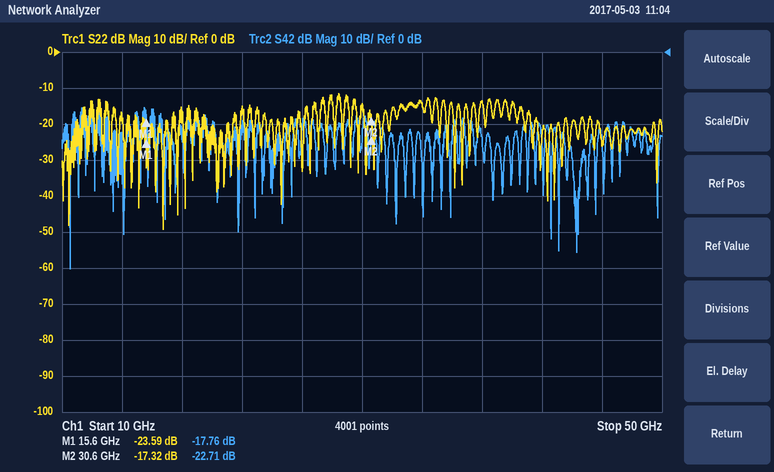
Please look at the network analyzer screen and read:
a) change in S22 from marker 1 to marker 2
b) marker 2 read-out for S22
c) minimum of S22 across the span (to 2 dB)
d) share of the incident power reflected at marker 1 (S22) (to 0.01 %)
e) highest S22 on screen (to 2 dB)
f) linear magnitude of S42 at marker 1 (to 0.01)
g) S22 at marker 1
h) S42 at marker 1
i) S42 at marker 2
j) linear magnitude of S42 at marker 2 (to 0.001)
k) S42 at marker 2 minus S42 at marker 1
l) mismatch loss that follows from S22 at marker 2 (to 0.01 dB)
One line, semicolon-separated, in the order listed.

6.27 dB; -17.32 dB; -50 dB; 0.44 %; -12 dB; 0.13; -23.59 dB; -17.76 dB; -22.71 dB; 0.073; -4.95 dB; 0.08 dB
